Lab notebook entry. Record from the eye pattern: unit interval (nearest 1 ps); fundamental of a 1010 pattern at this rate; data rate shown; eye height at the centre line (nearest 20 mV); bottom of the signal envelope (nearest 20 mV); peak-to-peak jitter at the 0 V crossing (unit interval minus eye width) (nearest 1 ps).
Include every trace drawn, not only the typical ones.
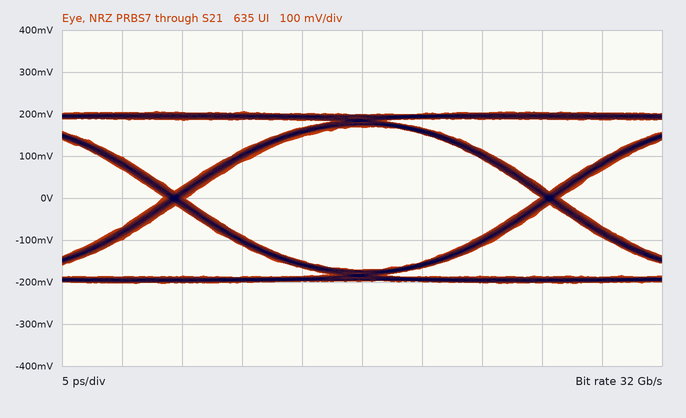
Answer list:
31 ps
16 GHz
32 Gb/s
340 mV
-200 mV
2 ps
